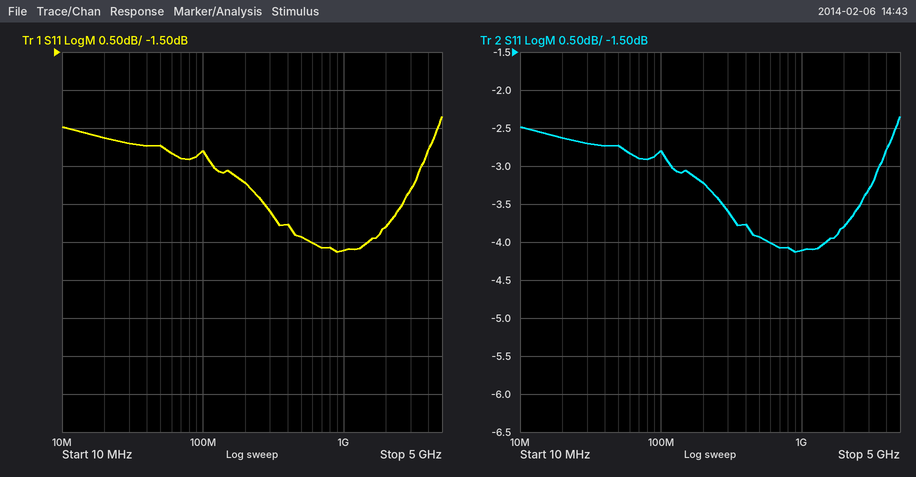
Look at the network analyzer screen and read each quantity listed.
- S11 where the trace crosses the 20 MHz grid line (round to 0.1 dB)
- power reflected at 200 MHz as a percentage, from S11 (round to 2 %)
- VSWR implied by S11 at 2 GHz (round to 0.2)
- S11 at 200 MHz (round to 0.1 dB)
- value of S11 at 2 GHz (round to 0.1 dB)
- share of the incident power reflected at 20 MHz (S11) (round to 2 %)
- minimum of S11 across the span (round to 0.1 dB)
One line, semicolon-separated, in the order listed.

-2.6 dB; 48 %; 4.6; -3.2 dB; -3.8 dB; 54 %; -4.1 dB
